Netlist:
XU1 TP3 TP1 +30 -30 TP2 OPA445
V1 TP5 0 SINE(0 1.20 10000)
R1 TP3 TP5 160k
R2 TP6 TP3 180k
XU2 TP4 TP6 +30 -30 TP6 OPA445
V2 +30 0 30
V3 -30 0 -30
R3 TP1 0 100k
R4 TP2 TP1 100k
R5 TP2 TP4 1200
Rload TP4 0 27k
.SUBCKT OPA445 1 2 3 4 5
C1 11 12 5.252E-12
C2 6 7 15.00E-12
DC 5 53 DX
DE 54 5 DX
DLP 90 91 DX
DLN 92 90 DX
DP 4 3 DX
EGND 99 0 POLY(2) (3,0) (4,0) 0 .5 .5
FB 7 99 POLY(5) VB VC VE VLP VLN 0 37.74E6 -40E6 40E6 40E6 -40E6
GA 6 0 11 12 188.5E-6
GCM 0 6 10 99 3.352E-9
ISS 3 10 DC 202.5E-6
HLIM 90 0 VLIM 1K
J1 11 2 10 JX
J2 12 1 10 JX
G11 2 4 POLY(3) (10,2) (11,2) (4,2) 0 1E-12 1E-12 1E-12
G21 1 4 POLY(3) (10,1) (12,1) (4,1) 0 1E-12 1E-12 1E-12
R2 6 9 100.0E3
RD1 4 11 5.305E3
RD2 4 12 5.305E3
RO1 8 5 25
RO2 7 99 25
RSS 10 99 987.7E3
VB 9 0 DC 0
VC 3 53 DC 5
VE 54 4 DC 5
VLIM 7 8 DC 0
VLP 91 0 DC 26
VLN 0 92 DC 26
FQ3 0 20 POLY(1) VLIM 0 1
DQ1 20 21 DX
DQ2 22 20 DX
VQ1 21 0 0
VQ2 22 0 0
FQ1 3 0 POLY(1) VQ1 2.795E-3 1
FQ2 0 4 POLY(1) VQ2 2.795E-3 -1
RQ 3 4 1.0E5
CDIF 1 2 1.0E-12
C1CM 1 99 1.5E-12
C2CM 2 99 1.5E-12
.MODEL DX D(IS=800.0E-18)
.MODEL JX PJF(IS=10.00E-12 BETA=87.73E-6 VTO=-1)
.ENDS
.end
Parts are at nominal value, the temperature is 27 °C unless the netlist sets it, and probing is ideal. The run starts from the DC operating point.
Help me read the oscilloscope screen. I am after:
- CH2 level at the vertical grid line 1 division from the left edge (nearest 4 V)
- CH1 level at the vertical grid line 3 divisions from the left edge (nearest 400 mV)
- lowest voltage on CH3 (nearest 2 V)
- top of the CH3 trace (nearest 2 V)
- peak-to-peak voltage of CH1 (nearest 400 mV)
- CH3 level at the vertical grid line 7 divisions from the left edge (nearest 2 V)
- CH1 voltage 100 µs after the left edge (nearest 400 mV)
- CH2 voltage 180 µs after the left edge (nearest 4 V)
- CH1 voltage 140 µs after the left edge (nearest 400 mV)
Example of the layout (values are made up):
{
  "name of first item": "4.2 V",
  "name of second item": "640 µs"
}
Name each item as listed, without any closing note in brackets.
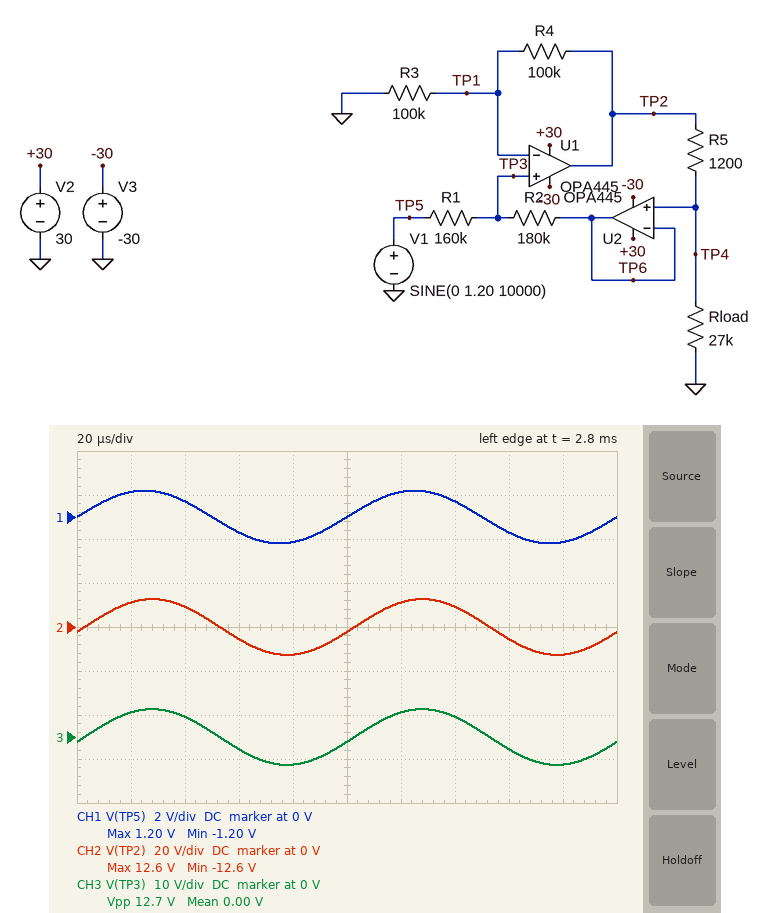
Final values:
{
  "CH2 level at the vertical grid line 1 division from the left edge": "12 V",
  "CH1 level at the vertical grid line 3 divisions from the left edge": "-800 mV",
  "lowest voltage on CH3": "-6 V",
  "top of the CH3 trace": "6 V",
  "peak-to-peak voltage of CH1": "2.4 V",
  "CH3 level at the vertical grid line 7 divisions from the left edge": "4 V",
  "CH1 voltage 100 µs after the left edge": "0 V",
  "CH2 voltage 180 µs after the left edge": "-12 V",
  "CH1 voltage 140 µs after the left edge": "800 mV"
}
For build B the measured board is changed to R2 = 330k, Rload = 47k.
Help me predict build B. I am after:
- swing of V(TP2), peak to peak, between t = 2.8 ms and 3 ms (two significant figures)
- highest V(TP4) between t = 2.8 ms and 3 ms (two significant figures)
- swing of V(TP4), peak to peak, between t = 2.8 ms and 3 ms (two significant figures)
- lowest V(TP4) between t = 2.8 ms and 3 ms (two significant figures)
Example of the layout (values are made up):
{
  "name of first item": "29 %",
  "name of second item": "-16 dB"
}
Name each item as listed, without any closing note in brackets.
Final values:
{
  "swing of V(TP2), peak to peak, between t = 2.8 ms and 3 ms": "8.9 V",
  "highest V(TP4) between t = 2.8 ms and 3 ms": "4.3 V",
  "swing of V(TP4), peak to peak, between t = 2.8 ms and 3 ms": "8.7 V",
  "lowest V(TP4) between t = 2.8 ms and 3 ms": "-4.3 V"
}
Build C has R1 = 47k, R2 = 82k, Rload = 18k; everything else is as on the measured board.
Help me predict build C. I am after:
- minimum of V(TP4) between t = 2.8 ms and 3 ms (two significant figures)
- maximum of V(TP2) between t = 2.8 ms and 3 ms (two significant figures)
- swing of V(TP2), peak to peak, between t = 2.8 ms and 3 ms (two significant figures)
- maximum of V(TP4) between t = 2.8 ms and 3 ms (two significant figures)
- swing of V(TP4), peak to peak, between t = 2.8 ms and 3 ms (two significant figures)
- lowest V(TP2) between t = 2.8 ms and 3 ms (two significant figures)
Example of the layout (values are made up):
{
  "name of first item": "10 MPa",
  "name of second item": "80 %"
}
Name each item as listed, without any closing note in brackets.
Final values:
{
  "minimum of V(TP4) between t = 2.8 ms and 3 ms": "-4.5 V",
  "maximum of V(TP2) between t = 2.8 ms and 3 ms": "4.8 V",
  "swing of V(TP2), peak to peak, between t = 2.8 ms and 3 ms": "9.6 V",
  "maximum of V(TP4) between t = 2.8 ms and 3 ms": "4.5 V",
  "swing of V(TP4), peak to peak, between t = 2.8 ms and 3 ms": "9.0 V",
  "lowest V(TP2) between t = 2.8 ms and 3 ms": "-4.8 V"
}
